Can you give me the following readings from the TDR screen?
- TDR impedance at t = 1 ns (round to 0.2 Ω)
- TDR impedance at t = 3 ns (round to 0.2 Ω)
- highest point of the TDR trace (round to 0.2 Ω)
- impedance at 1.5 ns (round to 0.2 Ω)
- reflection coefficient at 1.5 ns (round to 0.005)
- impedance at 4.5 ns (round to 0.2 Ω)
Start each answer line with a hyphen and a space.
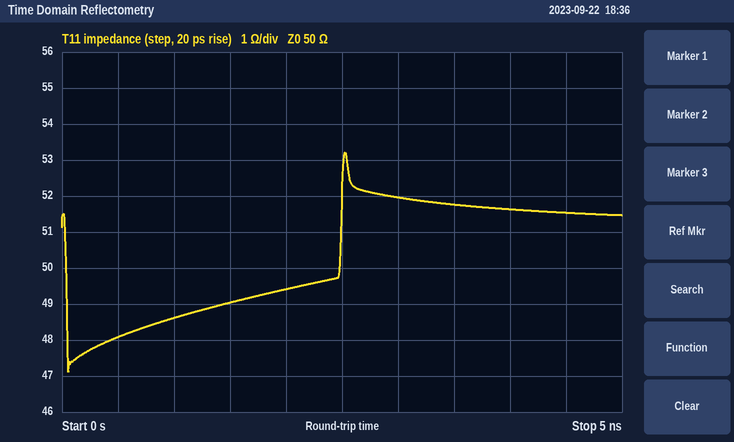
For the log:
- 48.6 Ω
- 52.0 Ω
- 53.2 Ω
- 49.0 Ω
- -0.010
- 51.6 Ω
